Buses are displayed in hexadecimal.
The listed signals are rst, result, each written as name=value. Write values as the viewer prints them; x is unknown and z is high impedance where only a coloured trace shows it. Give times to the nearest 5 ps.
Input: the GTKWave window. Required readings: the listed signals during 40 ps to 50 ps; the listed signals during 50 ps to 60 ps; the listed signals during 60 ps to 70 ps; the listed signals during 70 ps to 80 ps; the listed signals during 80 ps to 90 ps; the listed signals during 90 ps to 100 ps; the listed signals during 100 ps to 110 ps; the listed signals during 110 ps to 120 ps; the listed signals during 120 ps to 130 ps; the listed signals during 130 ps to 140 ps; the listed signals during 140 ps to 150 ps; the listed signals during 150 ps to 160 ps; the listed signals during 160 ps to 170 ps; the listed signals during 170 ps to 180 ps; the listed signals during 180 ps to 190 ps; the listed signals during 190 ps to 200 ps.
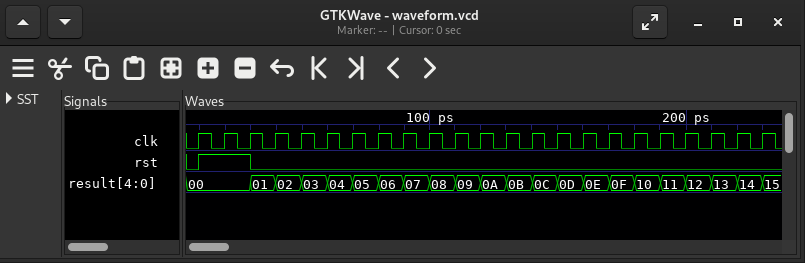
rst=0, result=02
rst=0, result=03
rst=0, result=04
rst=0, result=05
rst=0, result=06
rst=0, result=07
rst=0, result=08
rst=0, result=09
rst=0, result=0A
rst=0, result=0B
rst=0, result=0C
rst=0, result=0D
rst=0, result=0E
rst=0, result=0F
rst=0, result=10
rst=0, result=11
